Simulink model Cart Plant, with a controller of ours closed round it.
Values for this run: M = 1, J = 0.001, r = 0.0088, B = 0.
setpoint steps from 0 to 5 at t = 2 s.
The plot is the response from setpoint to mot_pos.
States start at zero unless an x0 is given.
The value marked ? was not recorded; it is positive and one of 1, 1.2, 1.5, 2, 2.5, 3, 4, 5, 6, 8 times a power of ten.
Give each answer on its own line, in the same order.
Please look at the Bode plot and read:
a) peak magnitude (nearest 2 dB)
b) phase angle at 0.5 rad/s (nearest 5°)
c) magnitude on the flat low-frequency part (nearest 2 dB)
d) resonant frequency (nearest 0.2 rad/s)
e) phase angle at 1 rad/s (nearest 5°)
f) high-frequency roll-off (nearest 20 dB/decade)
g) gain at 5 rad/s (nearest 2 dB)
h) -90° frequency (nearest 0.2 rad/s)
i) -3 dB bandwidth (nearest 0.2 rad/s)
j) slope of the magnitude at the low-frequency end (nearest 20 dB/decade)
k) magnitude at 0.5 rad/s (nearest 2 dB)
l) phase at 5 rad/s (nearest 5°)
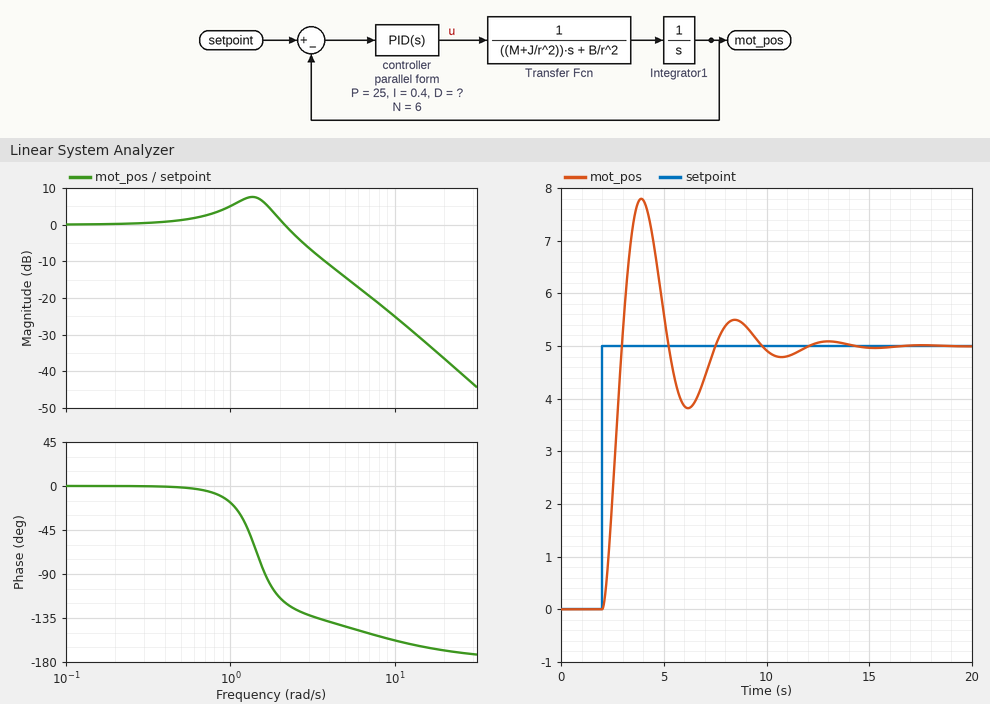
8 dB
0°
0 dB
1.4 rad/s
-15°
-40 dB/decade
-14 dB
1.6 rad/s
2.4 rad/s
0 dB/decade
2 dB
-145°
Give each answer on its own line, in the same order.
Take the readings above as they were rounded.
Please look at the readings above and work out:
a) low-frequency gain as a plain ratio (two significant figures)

1.0
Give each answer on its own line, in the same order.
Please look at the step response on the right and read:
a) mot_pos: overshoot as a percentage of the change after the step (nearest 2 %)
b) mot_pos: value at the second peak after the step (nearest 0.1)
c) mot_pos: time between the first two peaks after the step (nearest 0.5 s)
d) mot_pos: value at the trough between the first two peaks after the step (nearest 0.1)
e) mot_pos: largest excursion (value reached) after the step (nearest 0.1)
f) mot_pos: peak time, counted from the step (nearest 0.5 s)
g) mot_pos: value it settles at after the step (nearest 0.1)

56 %
5.5
4.5 s
3.8
7.8
2.0 s
5.0
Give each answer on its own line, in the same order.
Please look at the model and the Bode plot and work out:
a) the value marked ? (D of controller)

10
